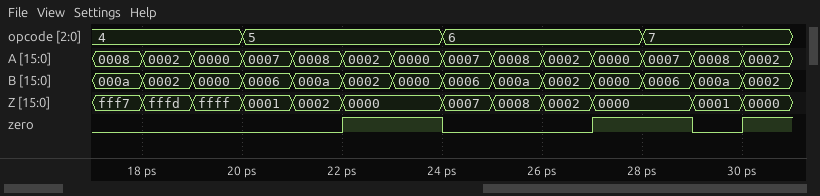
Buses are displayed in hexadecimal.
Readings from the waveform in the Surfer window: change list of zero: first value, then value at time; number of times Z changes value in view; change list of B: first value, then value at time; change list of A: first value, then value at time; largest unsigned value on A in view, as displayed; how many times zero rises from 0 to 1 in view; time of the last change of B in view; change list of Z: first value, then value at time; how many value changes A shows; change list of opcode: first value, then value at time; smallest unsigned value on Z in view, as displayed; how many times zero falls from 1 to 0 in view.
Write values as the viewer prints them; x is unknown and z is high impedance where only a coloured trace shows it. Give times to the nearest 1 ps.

0, 1 at 22 ps, 0 at 24 ps, 1 at 27 ps, 0 at 29 ps, 1 at 30 ps
11
000a, 0002 at 18 ps, 0000 at 19 ps, 0006 at 20 ps, 000a at 21 ps, 0002 at 22 ps, 0000 at 23 ps, 0006 at 24 ps, 000a at 25 ps, 0002 at 26 ps, 0000 at 27 ps, 0006 at 28 ps, 000a at 29 ps, 0002 at 30 ps
0008, 0002 at 18 ps, 0000 at 19 ps, 0007 at 20 ps, 0008 at 21 ps, 0002 at 22 ps, 0000 at 23 ps, 0007 at 24 ps, 0008 at 25 ps, 0002 at 26 ps, 0000 at 27 ps, 0007 at 28 ps, 0008 at 29 ps, 0002 at 30 ps
0008
3
30 ps
fff7, fffd at 18 ps, ffff at 19 ps, 0001 at 20 ps, 0002 at 21 ps, 0000 at 22 ps, 0007 at 24 ps, 0008 at 25 ps, 0002 at 26 ps, 0000 at 27 ps, 0001 at 29 ps, 0000 at 30 ps
13
4, 5 at 20 ps, 6 at 24 ps, 7 at 28 ps
0000
2
